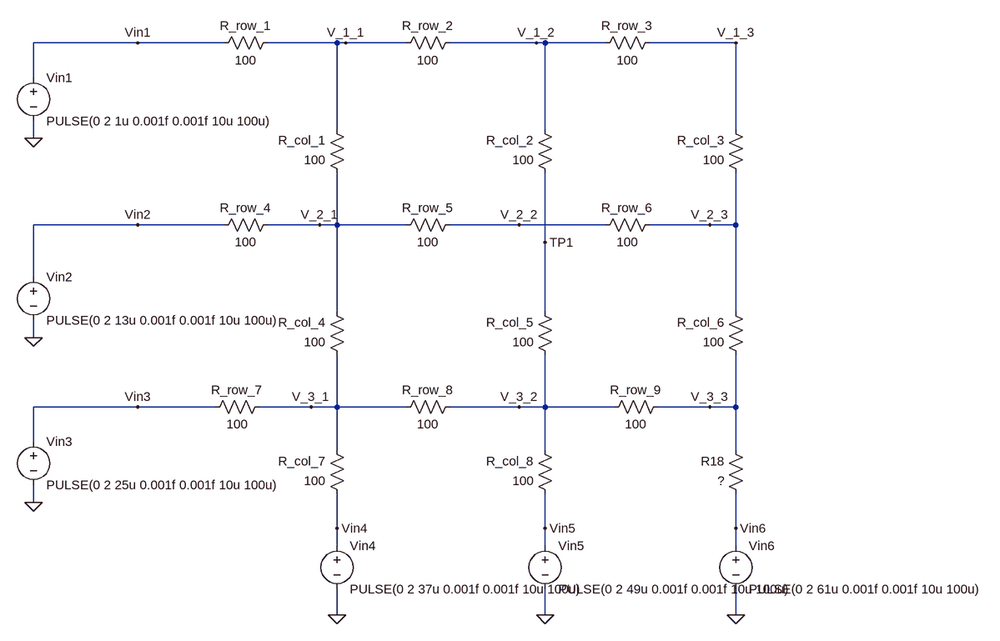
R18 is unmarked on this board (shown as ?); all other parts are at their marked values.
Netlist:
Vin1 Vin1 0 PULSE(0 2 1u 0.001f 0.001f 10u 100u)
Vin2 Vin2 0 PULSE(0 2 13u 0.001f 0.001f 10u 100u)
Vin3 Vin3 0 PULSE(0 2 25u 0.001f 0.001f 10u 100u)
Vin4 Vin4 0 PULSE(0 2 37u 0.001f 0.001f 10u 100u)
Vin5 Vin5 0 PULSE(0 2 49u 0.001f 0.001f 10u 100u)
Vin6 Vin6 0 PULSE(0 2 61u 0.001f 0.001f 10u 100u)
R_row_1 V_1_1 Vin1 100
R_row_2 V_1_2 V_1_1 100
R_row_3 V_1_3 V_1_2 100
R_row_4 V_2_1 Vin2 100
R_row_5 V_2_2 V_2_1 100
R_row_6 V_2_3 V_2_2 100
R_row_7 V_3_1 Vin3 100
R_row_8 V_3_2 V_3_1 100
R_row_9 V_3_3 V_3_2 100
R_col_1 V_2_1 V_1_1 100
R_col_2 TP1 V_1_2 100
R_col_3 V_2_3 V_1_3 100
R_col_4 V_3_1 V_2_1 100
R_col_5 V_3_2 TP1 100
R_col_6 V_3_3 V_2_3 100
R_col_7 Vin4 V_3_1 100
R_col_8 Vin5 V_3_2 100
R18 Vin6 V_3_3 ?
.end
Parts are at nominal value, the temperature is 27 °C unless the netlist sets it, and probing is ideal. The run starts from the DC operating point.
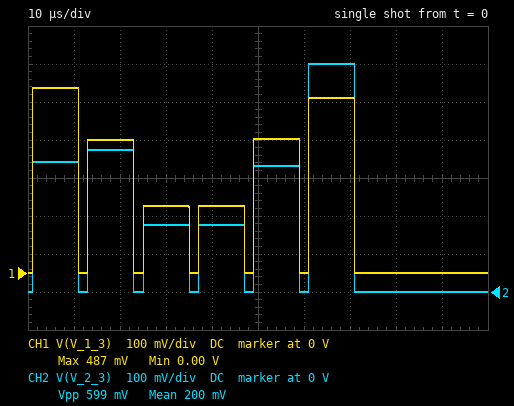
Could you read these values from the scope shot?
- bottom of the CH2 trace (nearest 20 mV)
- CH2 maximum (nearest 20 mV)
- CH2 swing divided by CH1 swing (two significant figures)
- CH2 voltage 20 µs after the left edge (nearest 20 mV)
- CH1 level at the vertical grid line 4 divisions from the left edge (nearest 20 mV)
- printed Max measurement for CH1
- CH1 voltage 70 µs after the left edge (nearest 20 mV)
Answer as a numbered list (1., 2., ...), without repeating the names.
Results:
1. 0 V
2. 600 mV
3. 1.2
4. 380 mV
5. 180 mV
6. 487 mV
7. 460 mV
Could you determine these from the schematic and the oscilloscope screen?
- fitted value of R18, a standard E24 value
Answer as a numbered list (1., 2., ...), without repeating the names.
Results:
1. 110 Ω
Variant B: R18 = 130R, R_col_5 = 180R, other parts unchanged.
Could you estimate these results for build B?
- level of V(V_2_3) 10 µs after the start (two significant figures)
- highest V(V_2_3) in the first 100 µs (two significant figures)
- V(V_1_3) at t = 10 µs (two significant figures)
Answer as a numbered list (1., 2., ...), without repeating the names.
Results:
1. 360 mV
2. 550 mV
3. 520 mV
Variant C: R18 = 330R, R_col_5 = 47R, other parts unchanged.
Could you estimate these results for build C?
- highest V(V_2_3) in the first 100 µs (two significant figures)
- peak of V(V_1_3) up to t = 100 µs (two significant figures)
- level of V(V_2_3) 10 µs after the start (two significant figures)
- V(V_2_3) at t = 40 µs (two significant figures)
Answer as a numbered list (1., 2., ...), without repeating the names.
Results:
1. 460 mV
2. 500 mV
3. 380 mV
4. 220 mV
